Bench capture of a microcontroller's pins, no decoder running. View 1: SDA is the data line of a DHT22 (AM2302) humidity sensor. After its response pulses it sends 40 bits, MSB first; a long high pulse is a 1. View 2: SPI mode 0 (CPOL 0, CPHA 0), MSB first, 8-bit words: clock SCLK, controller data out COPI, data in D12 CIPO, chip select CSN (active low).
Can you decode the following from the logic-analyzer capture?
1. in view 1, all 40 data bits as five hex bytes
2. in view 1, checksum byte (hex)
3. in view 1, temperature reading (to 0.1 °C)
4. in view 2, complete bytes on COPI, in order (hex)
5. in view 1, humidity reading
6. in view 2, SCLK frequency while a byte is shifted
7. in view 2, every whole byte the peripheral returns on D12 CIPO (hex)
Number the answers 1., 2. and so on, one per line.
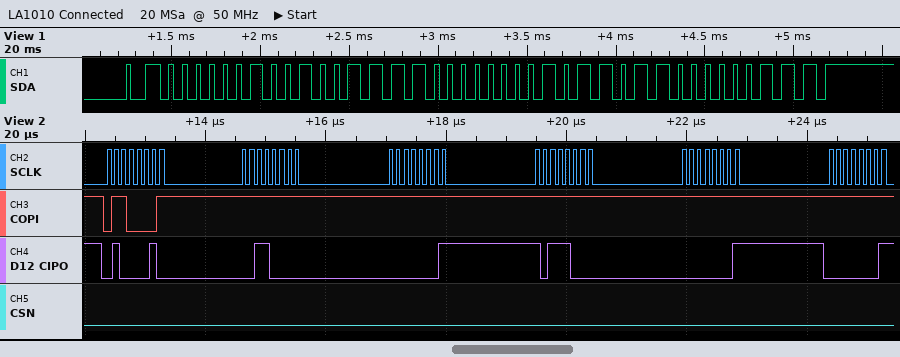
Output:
1. 02 4F 00 B6 07
2. 0x07
3. 18.2 °C
4. 61 FF FF FF FF FF
5. 59.1 %
6. 8 MHz
7. 42 30 01 B8 01 01
